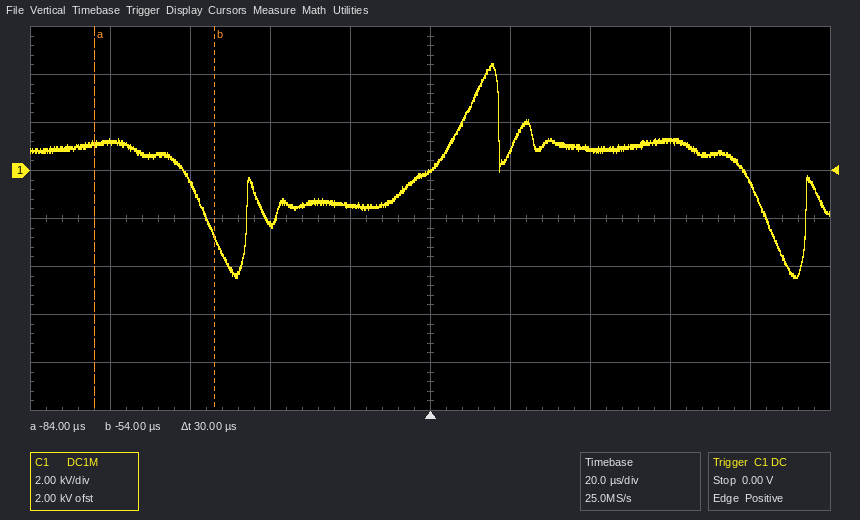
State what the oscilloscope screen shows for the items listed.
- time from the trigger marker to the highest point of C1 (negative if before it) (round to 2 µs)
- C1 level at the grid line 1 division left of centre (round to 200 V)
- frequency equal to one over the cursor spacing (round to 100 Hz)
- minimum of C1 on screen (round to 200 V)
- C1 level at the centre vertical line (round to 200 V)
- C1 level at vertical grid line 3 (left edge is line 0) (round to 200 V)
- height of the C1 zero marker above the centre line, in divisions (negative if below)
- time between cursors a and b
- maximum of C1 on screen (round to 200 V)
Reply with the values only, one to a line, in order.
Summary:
+16 µs
-1.4 kV
33.3 kHz
-4.4 kV
0.0 kV
-2.2 kV
+1.0 div
30 µs
4.4 kV
